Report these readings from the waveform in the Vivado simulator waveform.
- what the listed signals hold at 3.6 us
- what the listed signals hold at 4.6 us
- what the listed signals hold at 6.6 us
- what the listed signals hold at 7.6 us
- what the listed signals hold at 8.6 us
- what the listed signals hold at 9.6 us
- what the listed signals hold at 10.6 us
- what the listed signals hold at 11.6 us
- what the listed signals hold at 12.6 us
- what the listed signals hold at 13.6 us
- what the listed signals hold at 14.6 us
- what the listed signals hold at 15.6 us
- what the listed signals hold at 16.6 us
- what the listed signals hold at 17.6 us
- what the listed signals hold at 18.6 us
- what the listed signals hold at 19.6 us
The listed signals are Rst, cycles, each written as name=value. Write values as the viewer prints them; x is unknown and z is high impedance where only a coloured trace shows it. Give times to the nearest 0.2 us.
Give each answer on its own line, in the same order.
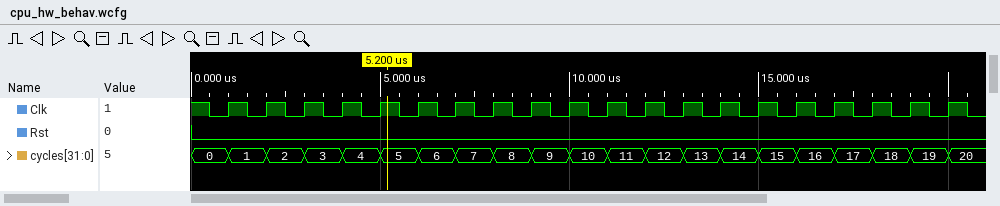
Rst=0, cycles=3
Rst=0, cycles=4
Rst=0, cycles=6
Rst=0, cycles=7
Rst=0, cycles=8
Rst=0, cycles=9
Rst=0, cycles=10
Rst=0, cycles=11
Rst=0, cycles=12
Rst=0, cycles=13
Rst=0, cycles=14
Rst=0, cycles=15
Rst=0, cycles=16
Rst=0, cycles=17
Rst=0, cycles=18
Rst=0, cycles=19
